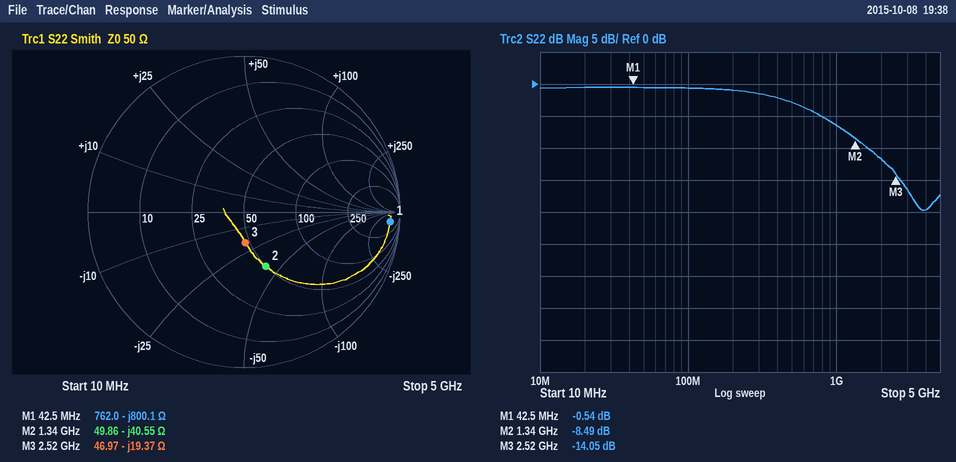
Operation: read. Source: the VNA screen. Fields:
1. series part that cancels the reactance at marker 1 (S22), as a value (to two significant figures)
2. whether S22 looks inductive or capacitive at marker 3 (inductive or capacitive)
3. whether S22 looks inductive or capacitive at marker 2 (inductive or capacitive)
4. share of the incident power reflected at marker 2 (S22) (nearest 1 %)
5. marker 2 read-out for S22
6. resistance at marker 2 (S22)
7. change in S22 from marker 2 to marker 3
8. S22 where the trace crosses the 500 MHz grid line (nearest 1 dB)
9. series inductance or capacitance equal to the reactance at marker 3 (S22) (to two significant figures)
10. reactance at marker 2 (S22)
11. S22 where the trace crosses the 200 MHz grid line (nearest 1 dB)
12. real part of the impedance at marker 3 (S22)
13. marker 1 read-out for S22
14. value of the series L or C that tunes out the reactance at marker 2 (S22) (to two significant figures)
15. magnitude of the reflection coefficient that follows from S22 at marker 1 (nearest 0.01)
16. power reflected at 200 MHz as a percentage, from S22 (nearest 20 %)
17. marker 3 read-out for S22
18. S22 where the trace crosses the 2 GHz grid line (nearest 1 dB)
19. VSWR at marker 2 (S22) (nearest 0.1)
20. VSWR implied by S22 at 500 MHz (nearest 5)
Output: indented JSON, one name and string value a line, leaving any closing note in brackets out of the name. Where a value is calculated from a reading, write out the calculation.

{
  "series part that cancels the reactance at marker 1 (S22), as a value": "L = 800.1 Ω/(2π × 42.5 MHz) ≈ 3.0 µH",
  "whether S22 looks inductive or capacitive at marker 3": "capacitive",
  "whether S22 looks inductive or capacitive at marker 2": "capacitive",
  "share of the incident power reflected at marker 2 (S22)": "10^(-8.49/10) ≈ 14 %",
  "marker 2 read-out for S22": "-8.49 dB",
  "resistance at marker 2": "49.86 Ω",
  "change in S22 from marker 2 to marker 3": "-14.05 − (-8.49) = -5.56 dB",
  "S22 where the trace crosses the 500 MHz grid line": "-3 dB",
  "series inductance or capacitance equal to the reactance at marker 3 (S22)": "C = 1/(2π × 2.52 GHz × 19.37 Ω) ≈ 3.3 pF",
  "reactance at marker 2": "-40.55 Ω",
  "S22 where the trace crosses the 200 MHz grid line": "-1 dB",
  "real part of the impedance at marker 3": "46.97 Ω",
  "marker 1 read-out for S22": "-0.54 dB",
  "value of the series L or C that tunes out the reactance at marker 2 (S22)": "L = 40.55 Ω/(2π × 1.34 GHz) ≈ 4.8 nH",
  "magnitude of the reflection coefficient that follows from S22 at marker 1": "10^(-0.54/20) ≈ 0.94",
  "power reflected at 200 MHz as a percentage, from S22": "10^(-1/10) ≈ 79.4 %, so 80 % to the nearest 20 %",
  "marker 3 read-out for S22": "-14.05 dB",
  "S22 where the trace crosses the 2 GHz grid line": "-12 dB",
  "VSWR at marker 2 (S22)": "2.2",
  "VSWR implied by S22 at 500 MHz": "|Γ| = 10^(-3/20) = 0.7079; VSWR = (1 + 0.7079)/(1 − 0.7079) ≈ 5.85, so 5 to the nearest 5"
}
